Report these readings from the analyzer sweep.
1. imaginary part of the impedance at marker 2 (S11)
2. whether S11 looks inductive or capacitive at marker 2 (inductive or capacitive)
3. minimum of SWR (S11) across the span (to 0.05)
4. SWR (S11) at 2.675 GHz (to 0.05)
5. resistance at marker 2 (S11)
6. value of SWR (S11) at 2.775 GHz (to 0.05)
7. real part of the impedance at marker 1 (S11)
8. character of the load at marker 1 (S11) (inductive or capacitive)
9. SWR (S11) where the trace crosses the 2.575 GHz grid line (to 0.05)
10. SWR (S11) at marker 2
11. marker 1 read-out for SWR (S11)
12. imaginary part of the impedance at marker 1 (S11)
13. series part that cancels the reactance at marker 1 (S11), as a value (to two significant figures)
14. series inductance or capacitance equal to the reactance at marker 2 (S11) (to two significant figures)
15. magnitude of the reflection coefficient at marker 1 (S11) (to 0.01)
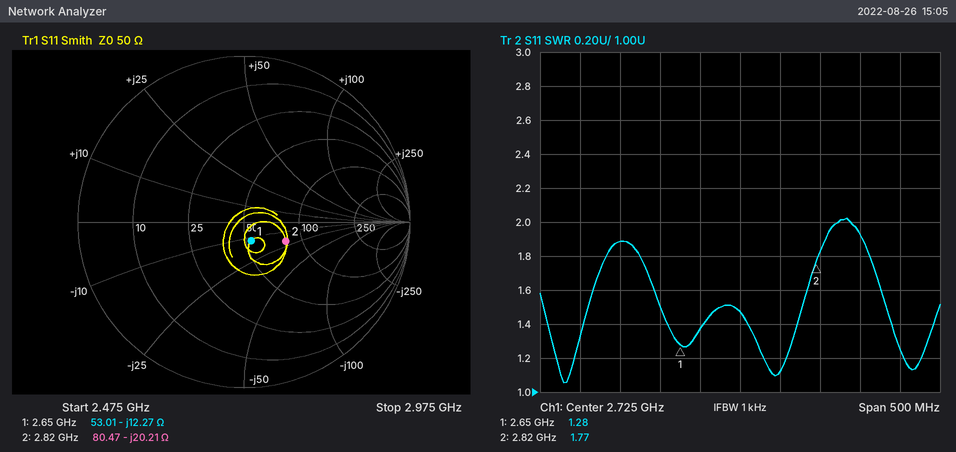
-20.21 Ω
capacitive
1.05
1.35
80.47 Ω
1.10
53.01 Ω
capacitive
1.90
1.77
1.28
-12.27 Ω
740 pH
2.8 pF
0.12
